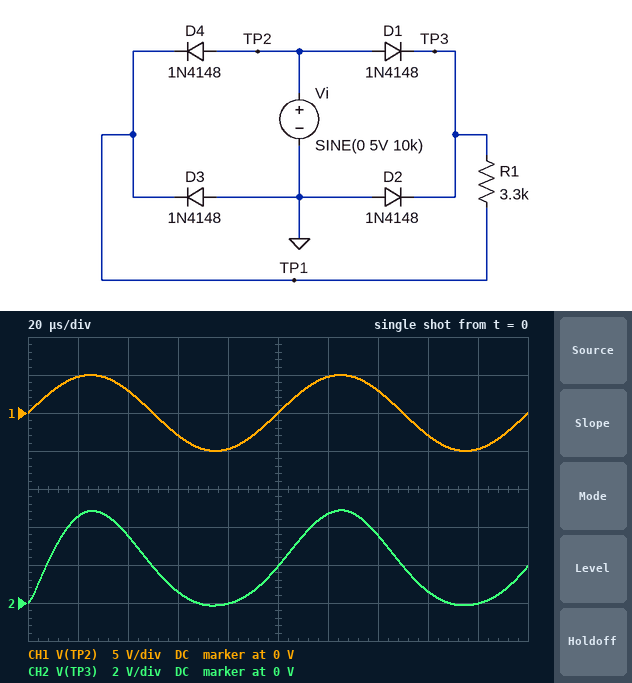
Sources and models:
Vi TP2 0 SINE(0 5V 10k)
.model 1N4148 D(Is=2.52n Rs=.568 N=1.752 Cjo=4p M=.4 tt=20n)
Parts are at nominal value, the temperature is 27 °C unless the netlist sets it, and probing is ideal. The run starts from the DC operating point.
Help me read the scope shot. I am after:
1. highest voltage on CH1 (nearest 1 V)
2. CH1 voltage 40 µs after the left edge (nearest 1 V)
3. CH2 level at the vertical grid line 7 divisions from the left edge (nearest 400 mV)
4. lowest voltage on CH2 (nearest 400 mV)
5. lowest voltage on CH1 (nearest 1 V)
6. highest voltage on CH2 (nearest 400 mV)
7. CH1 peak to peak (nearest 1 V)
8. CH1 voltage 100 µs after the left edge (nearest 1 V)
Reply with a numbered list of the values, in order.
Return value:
1. 5 V
2. 3 V
3. 3.6 V
4. 0 V
5. -5 V
6. 4.8 V
7. 10 V
8. 0 V
